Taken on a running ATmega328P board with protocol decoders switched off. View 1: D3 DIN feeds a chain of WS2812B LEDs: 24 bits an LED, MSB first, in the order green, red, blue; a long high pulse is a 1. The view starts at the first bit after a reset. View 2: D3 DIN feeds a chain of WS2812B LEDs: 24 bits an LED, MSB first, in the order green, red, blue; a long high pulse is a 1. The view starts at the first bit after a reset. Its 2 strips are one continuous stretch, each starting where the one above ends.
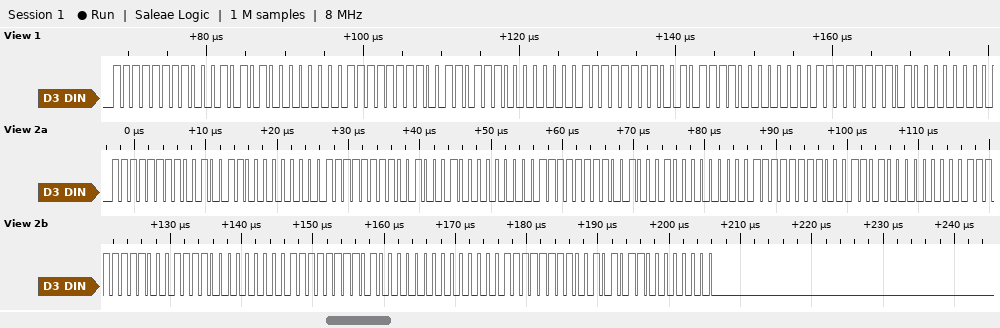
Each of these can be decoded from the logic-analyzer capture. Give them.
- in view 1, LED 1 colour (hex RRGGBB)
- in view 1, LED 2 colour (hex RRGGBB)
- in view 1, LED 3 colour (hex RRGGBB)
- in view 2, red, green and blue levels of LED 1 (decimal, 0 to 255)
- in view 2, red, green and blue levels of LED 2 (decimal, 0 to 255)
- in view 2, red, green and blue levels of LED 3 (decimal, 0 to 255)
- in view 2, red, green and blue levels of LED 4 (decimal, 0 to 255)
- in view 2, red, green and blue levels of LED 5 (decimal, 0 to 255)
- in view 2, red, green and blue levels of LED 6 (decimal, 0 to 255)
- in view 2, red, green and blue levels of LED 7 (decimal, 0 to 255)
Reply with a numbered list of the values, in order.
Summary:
1. #15FF00
2. #37FF00
3. #2FFF00
4. 38, 255, 0
5. 34, 255, 0
6. 34, 255, 0
7. 26, 255, 0
8. 30, 255, 0
9. 64, 255, 0
10. 43, 255, 0
